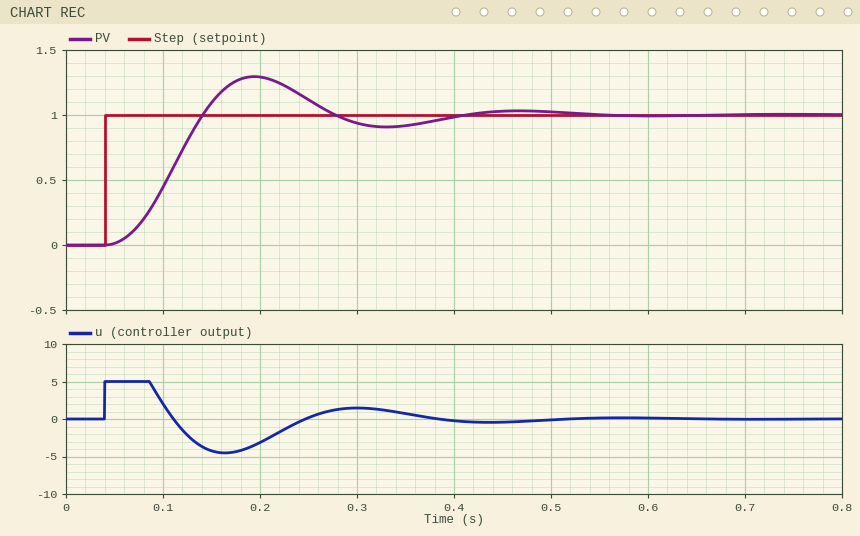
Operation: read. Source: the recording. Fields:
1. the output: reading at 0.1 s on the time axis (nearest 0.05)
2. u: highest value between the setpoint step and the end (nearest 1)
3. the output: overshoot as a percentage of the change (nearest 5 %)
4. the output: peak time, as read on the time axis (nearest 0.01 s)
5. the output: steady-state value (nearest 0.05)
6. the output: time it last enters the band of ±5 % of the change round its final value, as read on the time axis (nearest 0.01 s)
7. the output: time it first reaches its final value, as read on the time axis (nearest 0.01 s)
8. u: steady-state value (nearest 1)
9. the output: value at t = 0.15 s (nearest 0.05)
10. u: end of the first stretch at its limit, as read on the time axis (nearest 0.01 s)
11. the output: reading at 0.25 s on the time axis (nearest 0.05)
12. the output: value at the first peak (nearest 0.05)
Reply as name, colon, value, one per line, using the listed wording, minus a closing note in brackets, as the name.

the output: reading at 0.1 s on the time axis: 0.45
u: highest value between the setpoint step and the end: 5
the output: overshoot as a percentage of the change: 30 %
the output: peak time, as read on the time axis: 0.19 s
the output: steady-state value: 1.00
the output: time it last enters the band of ±5 % of the change round its final value, as read on the time axis: 0.38 s
the output: time it first reaches its final value, as read on the time axis: 0.14 s
u: steady-state value: 0
the output: value at t = 0.15 s: 1.10
u: end of the first stretch at its limit, as read on the time axis: 0.09 s
the output: reading at 0.25 s on the time axis: 1.10
the output: value at the first peak: 1.30
